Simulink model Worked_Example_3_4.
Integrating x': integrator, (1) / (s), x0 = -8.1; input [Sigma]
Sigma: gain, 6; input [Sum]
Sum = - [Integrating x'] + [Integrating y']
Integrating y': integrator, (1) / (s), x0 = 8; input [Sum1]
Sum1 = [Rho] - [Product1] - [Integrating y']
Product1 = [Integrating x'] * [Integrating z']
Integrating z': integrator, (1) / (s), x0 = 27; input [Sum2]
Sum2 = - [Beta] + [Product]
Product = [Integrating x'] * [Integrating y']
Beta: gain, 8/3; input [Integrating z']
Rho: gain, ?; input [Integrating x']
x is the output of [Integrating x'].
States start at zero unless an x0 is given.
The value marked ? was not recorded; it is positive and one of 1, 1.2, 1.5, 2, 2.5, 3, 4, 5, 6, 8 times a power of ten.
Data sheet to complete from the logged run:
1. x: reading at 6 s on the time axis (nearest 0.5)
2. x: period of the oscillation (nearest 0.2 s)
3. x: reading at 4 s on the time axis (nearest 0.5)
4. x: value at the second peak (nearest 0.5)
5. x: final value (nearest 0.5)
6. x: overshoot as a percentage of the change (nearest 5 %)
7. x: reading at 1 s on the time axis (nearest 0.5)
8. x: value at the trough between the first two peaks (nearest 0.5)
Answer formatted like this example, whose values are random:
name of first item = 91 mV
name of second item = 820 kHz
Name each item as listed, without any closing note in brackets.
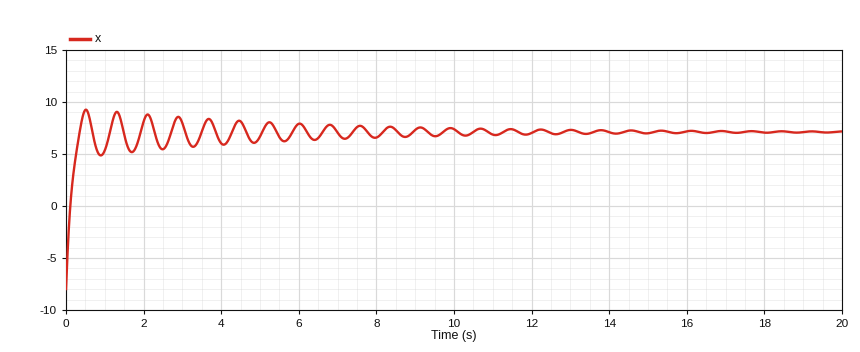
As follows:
x: reading at 6 s on the time axis = 8.0
x: period of the oscillation = 0.8 s
x: reading at 4 s on the time axis = 6.0
x: value at the second peak = 9.0
x: final value = 7.0
x: overshoot as a percentage of the change = 15 %
x: reading at 1 s on the time axis = 5.5
x: value at the trough between the first two peaks = 5.0
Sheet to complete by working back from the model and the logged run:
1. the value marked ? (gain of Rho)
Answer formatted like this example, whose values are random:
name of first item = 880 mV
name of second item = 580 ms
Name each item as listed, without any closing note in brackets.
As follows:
the value marked ? = 20
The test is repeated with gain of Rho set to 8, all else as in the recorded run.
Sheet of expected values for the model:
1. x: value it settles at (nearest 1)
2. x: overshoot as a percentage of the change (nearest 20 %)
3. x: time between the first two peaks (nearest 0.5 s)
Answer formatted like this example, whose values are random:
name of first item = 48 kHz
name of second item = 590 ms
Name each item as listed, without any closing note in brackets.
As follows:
x: value it settles at = -4
x: overshoot as a percentage of the change = 260 %
x: time between the first two peaks = 3.0 s
